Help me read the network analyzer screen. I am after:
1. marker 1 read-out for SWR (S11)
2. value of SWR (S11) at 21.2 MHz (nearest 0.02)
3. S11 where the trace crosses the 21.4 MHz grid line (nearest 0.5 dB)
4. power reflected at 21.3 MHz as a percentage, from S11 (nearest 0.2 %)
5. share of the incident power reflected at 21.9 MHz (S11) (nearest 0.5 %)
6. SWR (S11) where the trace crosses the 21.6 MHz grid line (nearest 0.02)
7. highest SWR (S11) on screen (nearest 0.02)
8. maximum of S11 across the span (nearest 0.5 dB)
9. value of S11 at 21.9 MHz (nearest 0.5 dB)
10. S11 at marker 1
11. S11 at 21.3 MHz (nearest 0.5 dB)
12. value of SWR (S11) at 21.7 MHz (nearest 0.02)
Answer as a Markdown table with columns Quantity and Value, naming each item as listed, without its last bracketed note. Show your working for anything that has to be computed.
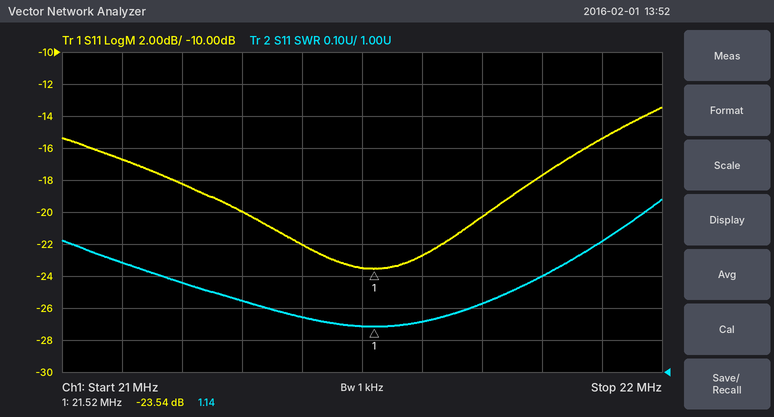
| Quantity | Value |
|---|---|
| marker 1 read-out for SWR | 1.14 |
| value of SWR (S11) at 21.2 MHz | 1.28 |
| S11 where the trace crosses the 21.4 MHz grid line | -22.0 dB |
| power reflected at 21.3 MHz as a percentage, from S11 | 10^(-20/10) ≈ 1.0 % |
| share of the incident power reflected at 21.9 MHz (S11) | 10^(-15.5/10) ≈ 2.82 %, so 3.0 % to the nearest 0.5 % |
| SWR (S11) where the trace crosses the 21.6 MHz grid line | 1.16 |
| highest SWR (S11) on screen | 1.54 |
| maximum of S11 across the span | -13.5 dB |
| value of S11 at 21.9 MHz | -15.5 dB |
| S11 at marker 1 | -23.54 dB |
| S11 at 21.3 MHz | -20.0 dB |
| value of SWR (S11) at 21.7 MHz | 1.22 |
